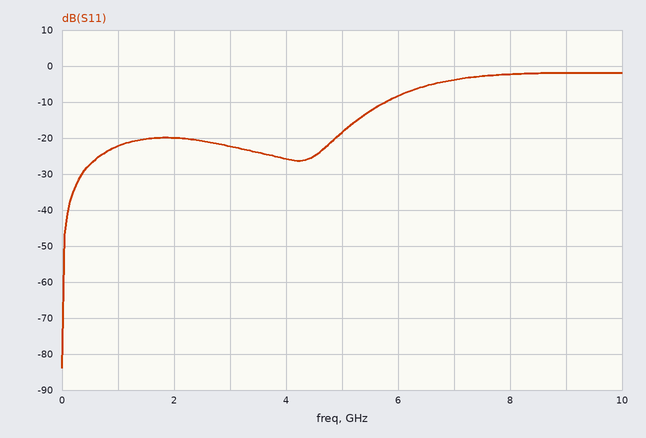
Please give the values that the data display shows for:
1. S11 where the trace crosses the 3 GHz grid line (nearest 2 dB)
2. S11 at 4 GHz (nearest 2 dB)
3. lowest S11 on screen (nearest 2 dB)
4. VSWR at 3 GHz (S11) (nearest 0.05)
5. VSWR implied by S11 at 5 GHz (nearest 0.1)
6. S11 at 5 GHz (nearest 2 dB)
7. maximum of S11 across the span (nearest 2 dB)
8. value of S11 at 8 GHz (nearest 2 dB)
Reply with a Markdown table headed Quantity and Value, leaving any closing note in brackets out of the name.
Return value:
| Quantity | Value |
|---|---|
| S11 where the trace crosses the 3 GHz grid line | -22 dB |
| S11 at 4 GHz | -26 dB |
| lowest S11 on screen | -84 dB |
| VSWR at 3 GHz (S11) | 1.15 |
| VSWR implied by S11 at 5 GHz | 1.3 |
| S11 at 5 GHz | -18 dB |
| maximum of S11 across the span | -2 dB |
| value of S11 at 8 GHz | -2 dB |
